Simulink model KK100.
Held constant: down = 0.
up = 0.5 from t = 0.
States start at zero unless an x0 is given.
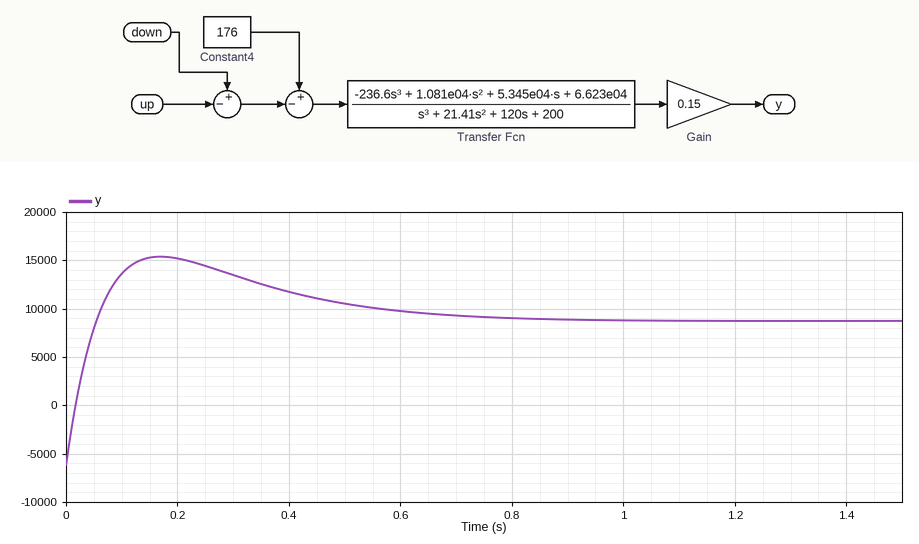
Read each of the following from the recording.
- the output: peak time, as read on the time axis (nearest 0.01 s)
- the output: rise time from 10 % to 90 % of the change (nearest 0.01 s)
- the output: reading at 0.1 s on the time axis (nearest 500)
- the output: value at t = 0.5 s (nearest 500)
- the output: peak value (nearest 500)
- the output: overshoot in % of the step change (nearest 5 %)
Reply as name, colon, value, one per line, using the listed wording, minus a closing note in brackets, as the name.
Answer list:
the output: peak time, as read on the time axis: 0.17 s
the output: rise time from 10 % to 90 % of the change: 0.04 s
the output: reading at 0.1 s on the time axis: 13500
the output: value at t = 0.5 s: 10500
the output: peak value: 15500
the output: overshoot in % of the step change: 45 %
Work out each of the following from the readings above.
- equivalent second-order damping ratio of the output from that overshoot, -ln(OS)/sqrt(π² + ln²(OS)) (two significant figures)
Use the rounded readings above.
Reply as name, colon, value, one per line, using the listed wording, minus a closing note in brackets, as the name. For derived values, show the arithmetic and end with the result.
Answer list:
equivalent second-order damping ratio of the output from that overshoot, -ln(OS)/sqrt(π² + ln²(OS)): ln(0.45) = -0.799; 0.799 / sqrt(9.870 + 0.638) = 0.25
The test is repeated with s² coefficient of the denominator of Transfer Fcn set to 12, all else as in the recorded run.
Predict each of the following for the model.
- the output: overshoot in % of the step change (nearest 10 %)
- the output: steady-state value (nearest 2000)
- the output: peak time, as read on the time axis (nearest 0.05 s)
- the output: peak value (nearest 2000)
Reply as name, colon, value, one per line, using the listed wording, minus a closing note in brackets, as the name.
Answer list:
the output: overshoot in % of the step change: 90 %
the output: steady-state value: 8000
the output: peak time, as read on the time axis: 0.15 s
the output: peak value: 22000
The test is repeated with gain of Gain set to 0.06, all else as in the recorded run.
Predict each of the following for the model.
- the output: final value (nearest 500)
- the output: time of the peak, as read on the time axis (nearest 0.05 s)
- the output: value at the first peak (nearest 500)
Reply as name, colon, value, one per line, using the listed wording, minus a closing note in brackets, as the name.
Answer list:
the output: final value: 3500
the output: time of the peak, as read on the time axis: 0.15 s
the output: value at the first peak: 6000
